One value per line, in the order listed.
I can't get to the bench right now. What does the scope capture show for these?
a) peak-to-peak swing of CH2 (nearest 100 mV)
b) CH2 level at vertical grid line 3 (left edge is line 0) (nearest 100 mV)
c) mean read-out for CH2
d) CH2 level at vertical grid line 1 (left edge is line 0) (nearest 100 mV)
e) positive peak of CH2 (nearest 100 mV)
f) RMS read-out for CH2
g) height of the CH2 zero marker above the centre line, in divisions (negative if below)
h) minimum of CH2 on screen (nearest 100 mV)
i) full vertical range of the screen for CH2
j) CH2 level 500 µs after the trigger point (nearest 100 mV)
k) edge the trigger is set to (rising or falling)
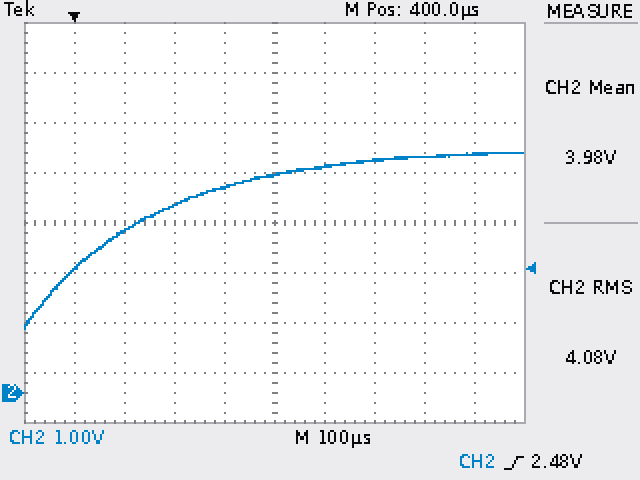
3.5 V
3.8 V
3.98 V
2.5 V
4.8 V
4.08 V
-3.4 div
1.3 V
8 V
4.5 V
rising
